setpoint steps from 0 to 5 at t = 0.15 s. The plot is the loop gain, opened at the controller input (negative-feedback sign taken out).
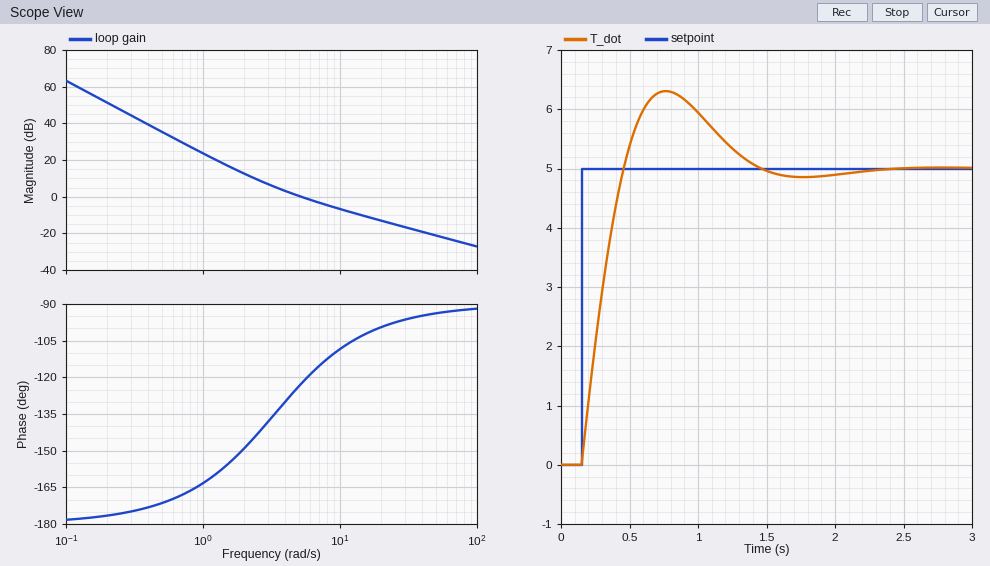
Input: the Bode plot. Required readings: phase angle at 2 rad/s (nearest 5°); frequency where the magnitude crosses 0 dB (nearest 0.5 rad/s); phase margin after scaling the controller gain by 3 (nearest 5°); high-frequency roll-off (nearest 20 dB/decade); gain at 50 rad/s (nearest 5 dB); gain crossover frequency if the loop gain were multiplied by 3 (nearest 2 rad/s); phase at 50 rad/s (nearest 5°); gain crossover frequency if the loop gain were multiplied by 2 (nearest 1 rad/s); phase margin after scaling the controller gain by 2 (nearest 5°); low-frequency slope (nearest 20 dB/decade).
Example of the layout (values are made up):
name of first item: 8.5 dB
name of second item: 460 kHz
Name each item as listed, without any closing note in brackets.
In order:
phase angle at 2 rad/s: -150°
frequency where the magnitude crosses 0 dB: 5.0 rad/s
phase margin after scaling the controller gain by 3: 75°
high-frequency roll-off: -20 dB/decade
gain at 50 rad/s: -20 dB
gain crossover frequency if the loop gain were multiplied by 3: 14 rad/s
phase at 50 rad/s: -95°
gain crossover frequency if the loop gain were multiplied by 2: 9 rad/s
phase margin after scaling the controller gain by 2: 70°
low-frequency slope: -40 dB/decade
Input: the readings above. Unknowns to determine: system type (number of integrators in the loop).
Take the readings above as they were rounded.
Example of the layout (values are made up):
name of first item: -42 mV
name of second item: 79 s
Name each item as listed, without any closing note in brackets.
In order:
system type: 2
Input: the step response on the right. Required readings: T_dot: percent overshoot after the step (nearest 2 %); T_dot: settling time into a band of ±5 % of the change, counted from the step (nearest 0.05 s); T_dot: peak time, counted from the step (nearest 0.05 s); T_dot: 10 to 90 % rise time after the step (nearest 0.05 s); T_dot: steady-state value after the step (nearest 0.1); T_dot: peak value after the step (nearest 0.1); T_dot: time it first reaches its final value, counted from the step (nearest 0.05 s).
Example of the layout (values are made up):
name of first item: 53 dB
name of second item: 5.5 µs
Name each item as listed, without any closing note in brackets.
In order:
T_dot: percent overshoot after the step: 26 %
T_dot: settling time into a band of ±5 % of the change, counted from the step: 1.15 s
T_dot: peak time, counted from the step: 0.60 s
T_dot: 10 to 90 % rise time after the step: 0.25 s
T_dot: steady-state value after the step: 5.0
T_dot: peak value after the step: 6.3
T_dot: time it first reaches its final value, counted from the step: 0.30 s
